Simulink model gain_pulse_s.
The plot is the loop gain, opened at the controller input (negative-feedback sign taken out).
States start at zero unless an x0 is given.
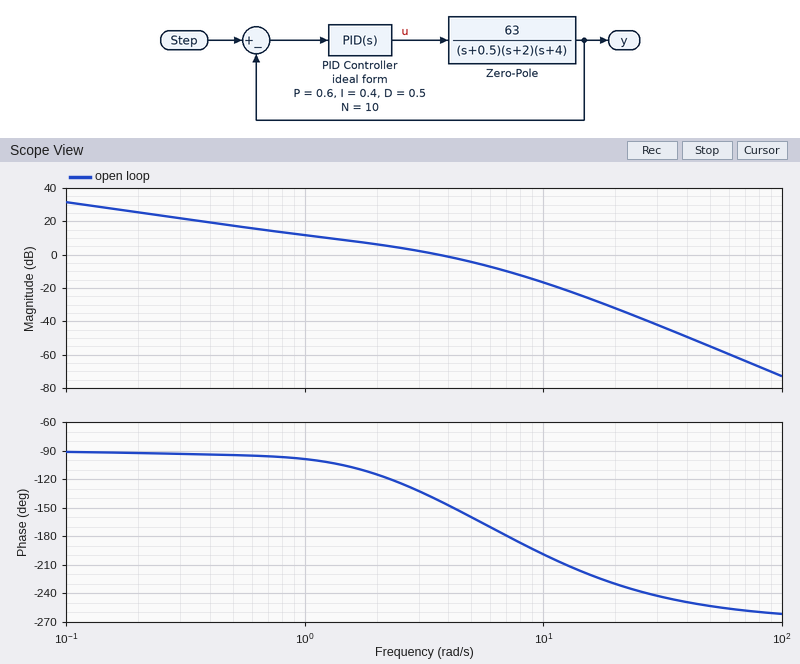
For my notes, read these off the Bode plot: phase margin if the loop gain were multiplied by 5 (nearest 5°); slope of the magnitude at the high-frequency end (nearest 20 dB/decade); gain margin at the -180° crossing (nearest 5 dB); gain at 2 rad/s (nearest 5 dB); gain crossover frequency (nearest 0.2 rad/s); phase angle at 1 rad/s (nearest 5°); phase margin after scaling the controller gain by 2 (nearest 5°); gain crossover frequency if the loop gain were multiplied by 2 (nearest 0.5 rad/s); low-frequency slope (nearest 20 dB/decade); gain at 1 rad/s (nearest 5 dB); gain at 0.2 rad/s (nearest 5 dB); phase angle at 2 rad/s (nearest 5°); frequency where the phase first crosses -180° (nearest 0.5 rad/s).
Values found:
-10°
-60 dB/decade
10 dB
5 dB
3.6 rad/s
-100°
15°
5.5 rad/s
-20 dB/decade
10 dB
25 dB
-115°
7.0 rad/s
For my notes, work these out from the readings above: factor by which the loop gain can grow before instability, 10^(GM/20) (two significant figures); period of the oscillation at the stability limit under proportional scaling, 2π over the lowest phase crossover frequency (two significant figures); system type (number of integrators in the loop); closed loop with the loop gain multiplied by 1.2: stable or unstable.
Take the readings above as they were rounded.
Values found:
3.2
0.90 s
1
stable
